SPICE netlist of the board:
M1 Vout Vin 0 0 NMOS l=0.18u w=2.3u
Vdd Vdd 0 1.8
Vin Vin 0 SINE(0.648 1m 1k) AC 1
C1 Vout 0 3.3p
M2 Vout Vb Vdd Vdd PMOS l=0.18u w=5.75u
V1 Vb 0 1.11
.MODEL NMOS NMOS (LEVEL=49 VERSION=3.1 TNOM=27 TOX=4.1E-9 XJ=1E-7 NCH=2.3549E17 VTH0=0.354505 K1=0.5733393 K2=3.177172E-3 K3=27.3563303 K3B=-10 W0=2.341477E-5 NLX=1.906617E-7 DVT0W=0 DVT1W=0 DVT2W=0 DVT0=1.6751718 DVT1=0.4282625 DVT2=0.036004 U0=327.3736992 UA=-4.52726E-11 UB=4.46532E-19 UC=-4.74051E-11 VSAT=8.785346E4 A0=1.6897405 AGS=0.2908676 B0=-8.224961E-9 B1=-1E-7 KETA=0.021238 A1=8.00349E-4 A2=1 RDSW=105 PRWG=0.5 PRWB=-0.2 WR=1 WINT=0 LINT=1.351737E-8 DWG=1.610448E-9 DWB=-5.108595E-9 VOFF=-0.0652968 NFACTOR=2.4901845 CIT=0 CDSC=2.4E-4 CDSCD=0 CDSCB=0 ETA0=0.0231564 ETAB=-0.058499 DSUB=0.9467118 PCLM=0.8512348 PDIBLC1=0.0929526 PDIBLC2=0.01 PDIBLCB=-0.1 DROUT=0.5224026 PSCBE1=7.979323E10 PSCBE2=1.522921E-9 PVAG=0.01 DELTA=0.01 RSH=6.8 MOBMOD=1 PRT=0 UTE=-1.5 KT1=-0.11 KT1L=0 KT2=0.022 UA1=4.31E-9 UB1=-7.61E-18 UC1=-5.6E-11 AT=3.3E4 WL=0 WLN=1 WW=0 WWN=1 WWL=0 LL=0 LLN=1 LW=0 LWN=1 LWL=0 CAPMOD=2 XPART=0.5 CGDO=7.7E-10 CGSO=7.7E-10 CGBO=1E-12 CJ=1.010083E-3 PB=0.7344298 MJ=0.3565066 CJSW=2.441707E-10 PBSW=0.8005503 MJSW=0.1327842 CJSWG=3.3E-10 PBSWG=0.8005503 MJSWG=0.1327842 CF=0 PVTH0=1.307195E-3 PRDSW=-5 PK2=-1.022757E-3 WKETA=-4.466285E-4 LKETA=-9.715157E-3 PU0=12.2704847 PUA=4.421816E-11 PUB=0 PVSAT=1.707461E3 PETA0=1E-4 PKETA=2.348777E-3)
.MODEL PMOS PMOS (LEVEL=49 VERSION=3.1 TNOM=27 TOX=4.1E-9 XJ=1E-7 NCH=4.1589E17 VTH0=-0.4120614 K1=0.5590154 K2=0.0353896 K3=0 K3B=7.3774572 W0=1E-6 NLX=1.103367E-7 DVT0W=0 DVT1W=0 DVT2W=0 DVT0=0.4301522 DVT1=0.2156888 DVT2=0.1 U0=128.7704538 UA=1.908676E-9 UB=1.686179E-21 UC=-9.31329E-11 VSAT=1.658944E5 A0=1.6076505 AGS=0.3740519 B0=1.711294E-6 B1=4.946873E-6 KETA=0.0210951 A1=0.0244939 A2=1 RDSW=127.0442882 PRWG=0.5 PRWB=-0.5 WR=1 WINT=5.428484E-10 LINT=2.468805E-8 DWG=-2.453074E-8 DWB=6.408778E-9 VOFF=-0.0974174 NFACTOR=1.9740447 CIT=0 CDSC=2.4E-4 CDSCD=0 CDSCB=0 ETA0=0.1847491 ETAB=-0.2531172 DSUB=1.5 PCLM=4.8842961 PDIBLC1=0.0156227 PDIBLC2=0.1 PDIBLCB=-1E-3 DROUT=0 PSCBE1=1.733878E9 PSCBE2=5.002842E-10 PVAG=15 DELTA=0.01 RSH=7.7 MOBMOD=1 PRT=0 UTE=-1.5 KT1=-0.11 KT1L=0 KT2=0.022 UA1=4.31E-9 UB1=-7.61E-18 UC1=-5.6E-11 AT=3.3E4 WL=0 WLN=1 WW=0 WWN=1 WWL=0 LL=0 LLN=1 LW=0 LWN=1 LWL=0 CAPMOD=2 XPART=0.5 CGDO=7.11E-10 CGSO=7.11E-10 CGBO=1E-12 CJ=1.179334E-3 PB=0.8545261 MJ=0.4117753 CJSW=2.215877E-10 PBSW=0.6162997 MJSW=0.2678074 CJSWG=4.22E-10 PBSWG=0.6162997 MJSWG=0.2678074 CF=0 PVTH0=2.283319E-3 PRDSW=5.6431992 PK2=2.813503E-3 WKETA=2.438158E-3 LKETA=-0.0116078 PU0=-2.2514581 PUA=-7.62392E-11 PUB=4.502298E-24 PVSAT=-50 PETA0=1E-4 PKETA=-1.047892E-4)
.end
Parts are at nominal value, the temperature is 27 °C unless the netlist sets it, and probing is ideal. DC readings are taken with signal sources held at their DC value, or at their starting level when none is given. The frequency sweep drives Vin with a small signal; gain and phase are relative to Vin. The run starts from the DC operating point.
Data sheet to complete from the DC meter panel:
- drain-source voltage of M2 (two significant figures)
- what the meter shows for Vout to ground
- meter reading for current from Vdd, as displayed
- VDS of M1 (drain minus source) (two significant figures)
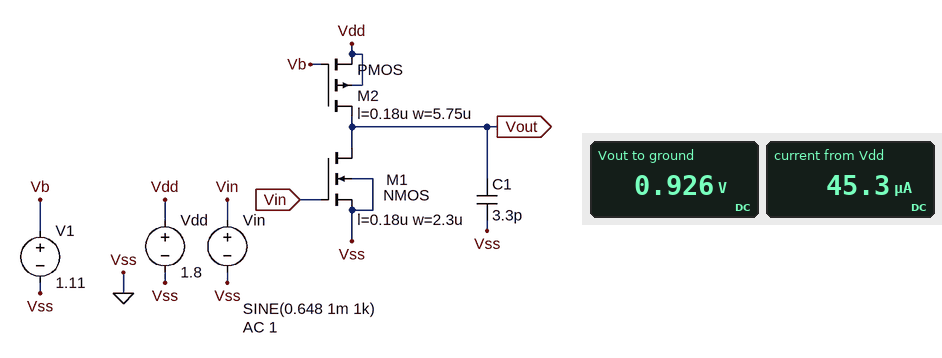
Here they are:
-870 mV
0.926 V
45.3 µA
930 mV
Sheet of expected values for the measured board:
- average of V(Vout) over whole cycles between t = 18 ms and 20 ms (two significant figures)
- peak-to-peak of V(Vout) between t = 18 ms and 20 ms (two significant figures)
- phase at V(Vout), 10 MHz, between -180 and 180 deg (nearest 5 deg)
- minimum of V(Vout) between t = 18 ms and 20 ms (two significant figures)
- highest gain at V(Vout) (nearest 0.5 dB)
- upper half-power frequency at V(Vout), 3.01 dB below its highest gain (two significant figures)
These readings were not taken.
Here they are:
930 mV
50 mV
95 deg
900 mV
28.0 dB
1.1 MHz
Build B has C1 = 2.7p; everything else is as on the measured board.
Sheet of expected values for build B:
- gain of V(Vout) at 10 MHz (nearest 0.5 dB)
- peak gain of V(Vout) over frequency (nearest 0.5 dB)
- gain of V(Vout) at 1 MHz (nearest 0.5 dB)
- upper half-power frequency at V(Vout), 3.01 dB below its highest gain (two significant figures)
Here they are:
10.5 dB
28.0 dB
26.0 dB
1.3 MHz
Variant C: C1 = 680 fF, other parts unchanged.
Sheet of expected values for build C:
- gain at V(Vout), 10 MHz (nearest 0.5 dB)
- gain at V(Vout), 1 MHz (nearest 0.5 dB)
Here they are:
21.5 dB
28.0 dB
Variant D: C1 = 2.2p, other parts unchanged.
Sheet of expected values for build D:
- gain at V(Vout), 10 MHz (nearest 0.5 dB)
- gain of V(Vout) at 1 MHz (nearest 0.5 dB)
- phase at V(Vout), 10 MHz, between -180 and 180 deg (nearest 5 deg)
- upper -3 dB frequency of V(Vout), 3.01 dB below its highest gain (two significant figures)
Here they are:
12.0 dB
26.5 dB
100 deg
1.6 MHz
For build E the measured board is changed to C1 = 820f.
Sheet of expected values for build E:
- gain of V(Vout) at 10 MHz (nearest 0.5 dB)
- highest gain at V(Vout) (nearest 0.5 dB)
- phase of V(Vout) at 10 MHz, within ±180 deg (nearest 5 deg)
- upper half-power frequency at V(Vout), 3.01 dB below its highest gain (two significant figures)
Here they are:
20.0 dB
28.0 dB
115 deg
4.4 MHz
